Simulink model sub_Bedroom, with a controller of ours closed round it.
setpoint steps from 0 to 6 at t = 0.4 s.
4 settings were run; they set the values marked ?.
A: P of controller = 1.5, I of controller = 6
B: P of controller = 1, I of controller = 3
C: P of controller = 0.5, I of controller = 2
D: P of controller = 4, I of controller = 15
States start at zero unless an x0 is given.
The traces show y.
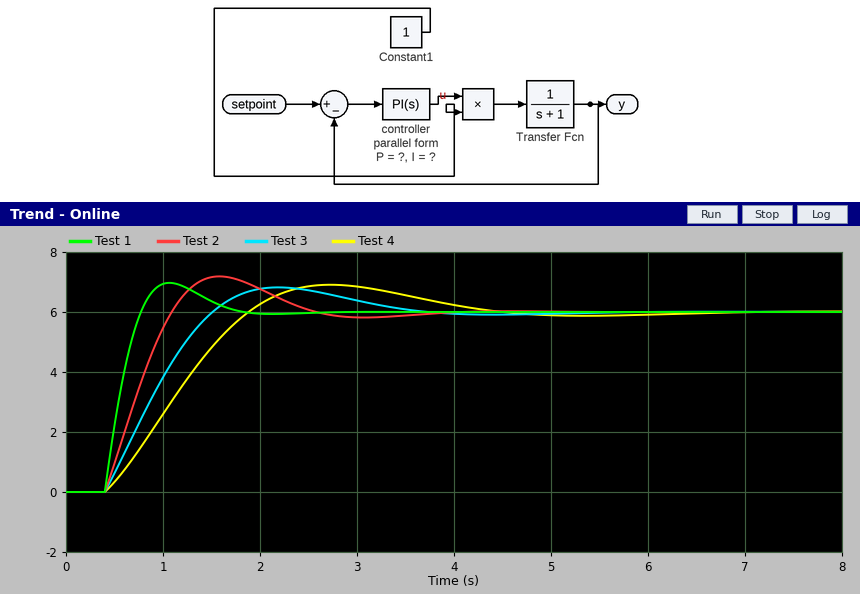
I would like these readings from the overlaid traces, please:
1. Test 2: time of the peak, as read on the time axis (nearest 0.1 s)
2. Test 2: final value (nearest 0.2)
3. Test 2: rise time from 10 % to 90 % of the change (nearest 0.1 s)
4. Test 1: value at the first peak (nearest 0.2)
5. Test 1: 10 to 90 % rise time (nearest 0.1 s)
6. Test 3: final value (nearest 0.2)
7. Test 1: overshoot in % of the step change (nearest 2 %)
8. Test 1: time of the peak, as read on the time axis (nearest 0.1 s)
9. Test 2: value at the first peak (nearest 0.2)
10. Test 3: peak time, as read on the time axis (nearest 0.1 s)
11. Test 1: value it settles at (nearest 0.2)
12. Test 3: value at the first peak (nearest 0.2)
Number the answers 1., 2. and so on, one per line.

1. 1.6 s
2. 6.0
3. 0.5 s
4. 7.0
5. 0.3 s
6. 6.0
7. 16 %
8. 1.1 s
9. 7.2
10. 2.2 s
11. 6.0
12. 6.8
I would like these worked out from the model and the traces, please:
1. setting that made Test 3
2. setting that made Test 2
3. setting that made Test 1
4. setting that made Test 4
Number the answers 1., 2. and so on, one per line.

1. B
2. A
3. D
4. C
